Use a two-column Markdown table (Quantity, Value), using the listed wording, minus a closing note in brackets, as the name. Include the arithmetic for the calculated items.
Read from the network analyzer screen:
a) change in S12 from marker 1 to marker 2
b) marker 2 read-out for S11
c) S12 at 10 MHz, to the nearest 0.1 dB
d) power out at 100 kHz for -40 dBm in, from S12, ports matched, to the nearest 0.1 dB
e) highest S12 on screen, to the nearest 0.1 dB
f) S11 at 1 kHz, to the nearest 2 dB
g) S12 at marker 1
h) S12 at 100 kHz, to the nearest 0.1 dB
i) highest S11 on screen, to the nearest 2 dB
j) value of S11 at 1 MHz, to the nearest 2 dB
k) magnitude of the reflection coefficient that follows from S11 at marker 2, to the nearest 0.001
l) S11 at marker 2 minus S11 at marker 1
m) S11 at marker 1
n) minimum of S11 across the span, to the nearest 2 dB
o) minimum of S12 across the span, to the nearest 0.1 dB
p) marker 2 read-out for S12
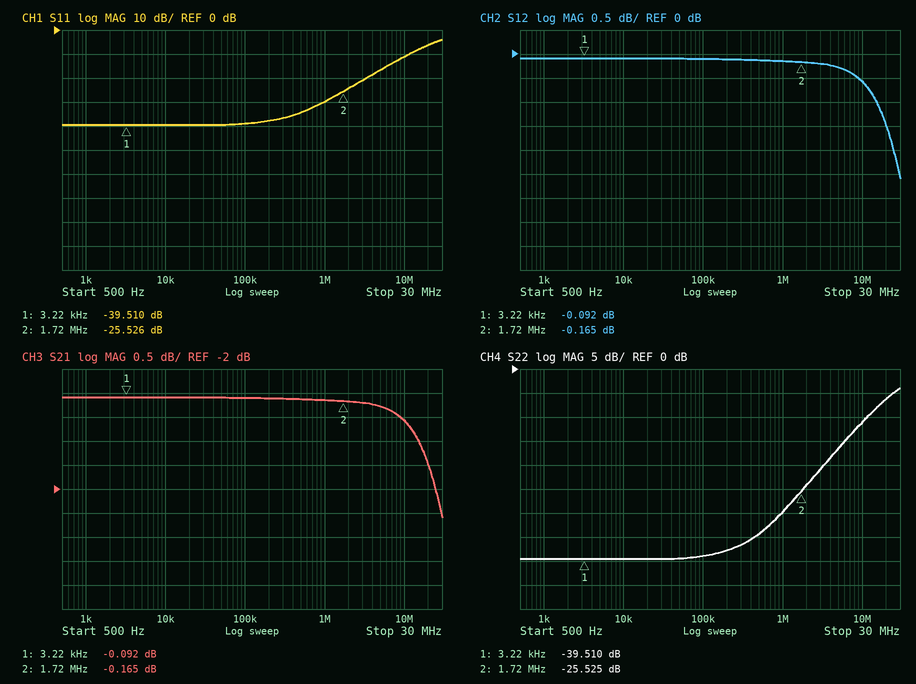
| Quantity | Value |
|---|---|
| change in S12 from marker 1 to marker 2 | -0.165 − (-0.092) = -0.073 dB |
| marker 2 read-out for S11 | -25.526 dB |
| S12 at 10 MHz, to the nearest 0.1 dB | -0.6 dB |
| power out at 100 kHz for -40 dBm in, from S12, ports matched, to the nearest 0.1 dB | -40 dBm + (-0.1 dB) = -40.1 dBm |
| highest S12 on screen, to the nearest 0.1 dB | -0.1 dB |
| S11 at 1 kHz, to the nearest 2 dB | -40 dB |
| S12 at marker 1 | -0.092 dB |
| S12 at 100 kHz, to the nearest 0.1 dB | -0.1 dB |
| highest S11 on screen, to the nearest 2 dB | -4 dB |
| value of S11 at 1 MHz, to the nearest 2 dB | -30 dB |
| magnitude of the reflection coefficient that follows from S11 at marker 2, to the nearest 0.001 | 10^(-25.526/20) ≈ 0.053 |
| S11 at marker 2 minus S11 at marker 1 | -25.526 − (-39.51) = 13.984 dB |
| S11 at marker 1 | -39.510 dB |
| minimum of S11 across the span, to the nearest 2 dB | -40 dB |
| minimum of S12 across the span, to the nearest 0.1 dB | -2.6 dB |
| marker 2 read-out for S12 | -0.165 dB |
